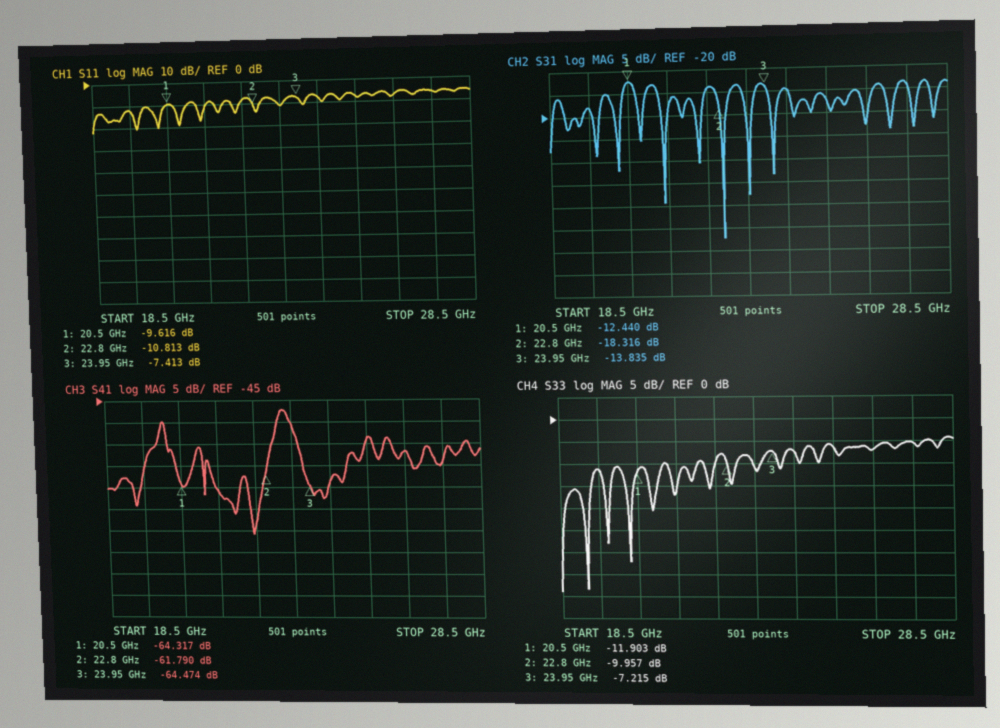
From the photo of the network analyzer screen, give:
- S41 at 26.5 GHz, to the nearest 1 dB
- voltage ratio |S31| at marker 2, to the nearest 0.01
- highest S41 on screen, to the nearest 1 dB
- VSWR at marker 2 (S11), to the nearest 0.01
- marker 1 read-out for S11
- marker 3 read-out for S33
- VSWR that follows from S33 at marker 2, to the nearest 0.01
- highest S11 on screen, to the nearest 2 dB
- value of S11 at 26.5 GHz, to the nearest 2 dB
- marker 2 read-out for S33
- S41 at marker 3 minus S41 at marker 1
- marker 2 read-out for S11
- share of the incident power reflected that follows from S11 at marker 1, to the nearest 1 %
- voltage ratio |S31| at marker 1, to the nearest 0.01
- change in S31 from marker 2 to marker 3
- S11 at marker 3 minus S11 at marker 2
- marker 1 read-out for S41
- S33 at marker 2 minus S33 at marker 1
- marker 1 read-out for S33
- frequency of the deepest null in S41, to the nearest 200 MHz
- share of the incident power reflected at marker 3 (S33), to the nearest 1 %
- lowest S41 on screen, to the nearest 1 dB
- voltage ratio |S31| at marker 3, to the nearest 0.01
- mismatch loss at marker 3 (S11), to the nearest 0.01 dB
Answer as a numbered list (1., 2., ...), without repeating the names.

1. -57 dB
2. 0.12
3. -47 dB
4. 1.81
5. -9.616 dB
6. -7.215 dB
7. 1.93
8. -6 dB
9. -8 dB
10. -9.957 dB
11. -0.157 dB
12. -10.813 dB
13. 11 %
14. 0.24
15. 4.481 dB
16. 3.400 dB
17. -64.317 dB
18. 1.946 dB
19. -11.903 dB
20. 22.4 GHz
21. 19 %
22. -76 dB
23. 0.20
24. 0.87 dB
